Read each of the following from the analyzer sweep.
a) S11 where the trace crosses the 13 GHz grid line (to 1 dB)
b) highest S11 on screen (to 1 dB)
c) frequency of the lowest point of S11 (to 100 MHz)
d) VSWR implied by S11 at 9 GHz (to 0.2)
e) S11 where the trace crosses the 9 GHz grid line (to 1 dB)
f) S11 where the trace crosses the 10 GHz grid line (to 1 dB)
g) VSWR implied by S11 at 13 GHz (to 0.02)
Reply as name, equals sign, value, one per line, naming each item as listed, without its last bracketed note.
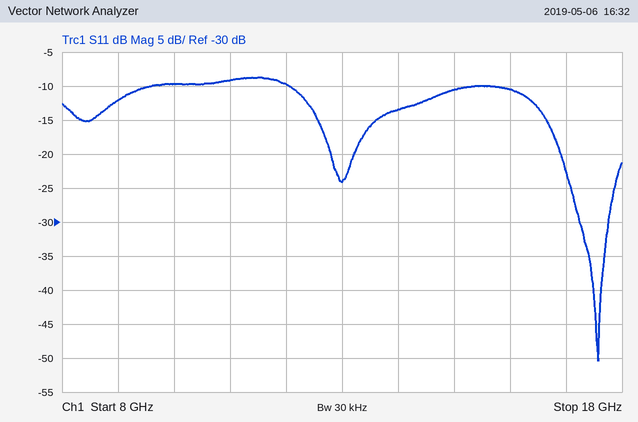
S11 where the trace crosses the 13 GHz grid line = -24 dB
highest S11 on screen = -9 dB
frequency of the lowest point of S11 = 17.6 GHz
VSWR implied by S11 at 9 GHz = 1.6
S11 where the trace crosses the 9 GHz grid line = -12 dB
S11 where the trace crosses the 10 GHz grid line = -10 dB
VSWR implied by S11 at 13 GHz = 1.14
